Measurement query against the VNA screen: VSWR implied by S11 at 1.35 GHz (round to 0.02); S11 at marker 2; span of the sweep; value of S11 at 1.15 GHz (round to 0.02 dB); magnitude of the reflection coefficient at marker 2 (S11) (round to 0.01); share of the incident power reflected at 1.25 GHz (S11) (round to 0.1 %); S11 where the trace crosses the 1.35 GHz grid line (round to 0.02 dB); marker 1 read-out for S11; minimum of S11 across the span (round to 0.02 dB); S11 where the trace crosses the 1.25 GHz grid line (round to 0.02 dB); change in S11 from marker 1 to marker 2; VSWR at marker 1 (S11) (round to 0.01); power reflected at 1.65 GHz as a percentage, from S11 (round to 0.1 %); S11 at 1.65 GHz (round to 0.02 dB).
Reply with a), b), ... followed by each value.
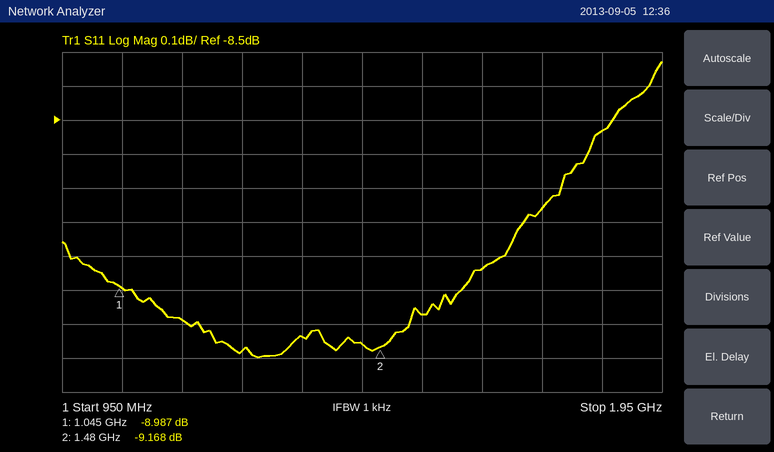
a) 2.08
b) -9.168 dB
c) 1 GHz
d) -9.08 dB
e) 0.35
f) 12.1 %
g) -9.14 dB
h) -8.987 dB
i) -9.20 dB
j) -9.18 dB
k) -0.181 dB
l) 2.10
m) 12.8 %
n) -8.94 dB
